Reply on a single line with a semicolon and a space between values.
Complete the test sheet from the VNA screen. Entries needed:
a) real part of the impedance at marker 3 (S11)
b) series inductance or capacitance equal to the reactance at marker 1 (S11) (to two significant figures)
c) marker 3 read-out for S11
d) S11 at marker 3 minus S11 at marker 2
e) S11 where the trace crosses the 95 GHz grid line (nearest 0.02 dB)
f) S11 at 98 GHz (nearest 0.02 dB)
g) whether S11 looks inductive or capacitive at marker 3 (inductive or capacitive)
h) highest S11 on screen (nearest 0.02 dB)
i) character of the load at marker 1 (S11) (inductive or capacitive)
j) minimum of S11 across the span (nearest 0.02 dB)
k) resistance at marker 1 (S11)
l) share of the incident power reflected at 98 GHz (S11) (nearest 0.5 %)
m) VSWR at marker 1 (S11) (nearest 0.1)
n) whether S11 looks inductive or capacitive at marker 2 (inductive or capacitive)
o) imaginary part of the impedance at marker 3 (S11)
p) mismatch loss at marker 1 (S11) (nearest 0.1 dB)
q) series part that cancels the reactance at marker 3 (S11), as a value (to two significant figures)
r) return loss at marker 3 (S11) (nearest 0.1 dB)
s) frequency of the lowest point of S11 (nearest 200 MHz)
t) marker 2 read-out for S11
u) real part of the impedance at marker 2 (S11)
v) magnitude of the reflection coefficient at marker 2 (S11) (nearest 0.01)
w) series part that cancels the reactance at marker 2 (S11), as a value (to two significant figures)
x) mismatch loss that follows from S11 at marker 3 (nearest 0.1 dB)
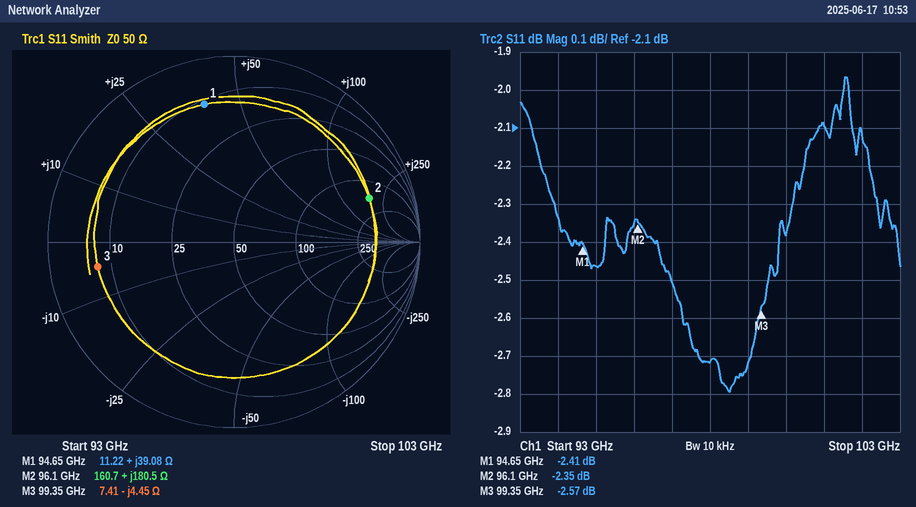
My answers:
7.41 Ω; 66 pH; -2.57 dB; -0.22 dB; -2.46 dB; -2.72 dB; capacitive; -1.96 dB; inductive; -2.80 dB; 11.22 Ω; 53.5 %; 7.3; inductive; -4.45 Ω; 3.7 dB; 7.1 pH; 2.6 dB; 98.6 GHz; -2.35 dB; 160.7 Ω; 0.76; 9.2 fF; 3.5 dB
